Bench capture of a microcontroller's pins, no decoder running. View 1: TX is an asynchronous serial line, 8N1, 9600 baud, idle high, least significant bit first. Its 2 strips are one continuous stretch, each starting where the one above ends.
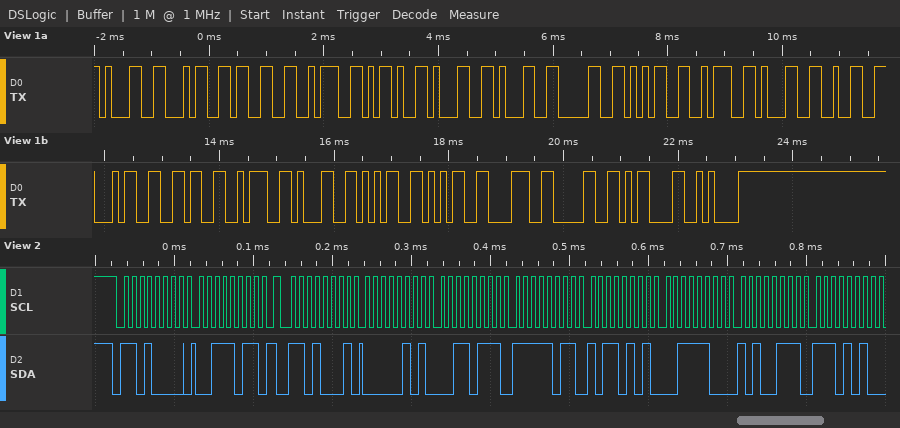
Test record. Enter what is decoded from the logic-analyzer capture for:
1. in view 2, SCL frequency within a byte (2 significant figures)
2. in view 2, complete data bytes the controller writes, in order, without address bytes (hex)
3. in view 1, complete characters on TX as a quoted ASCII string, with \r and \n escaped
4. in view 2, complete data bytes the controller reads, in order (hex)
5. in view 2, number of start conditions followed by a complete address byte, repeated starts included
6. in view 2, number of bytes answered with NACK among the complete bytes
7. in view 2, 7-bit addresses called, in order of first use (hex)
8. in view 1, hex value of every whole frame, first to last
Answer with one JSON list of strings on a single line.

["100 kHz", "3B", "\"143:-1105:1246:15580\\r\\n\"", "05 37 FB B5 3C A7 EA", "2", "0", "0x68", "31 34 33 3A 2D 31 31 30 35 3A 31 32 34 36 3A 31 35 35 38 30 0D 0A"]
